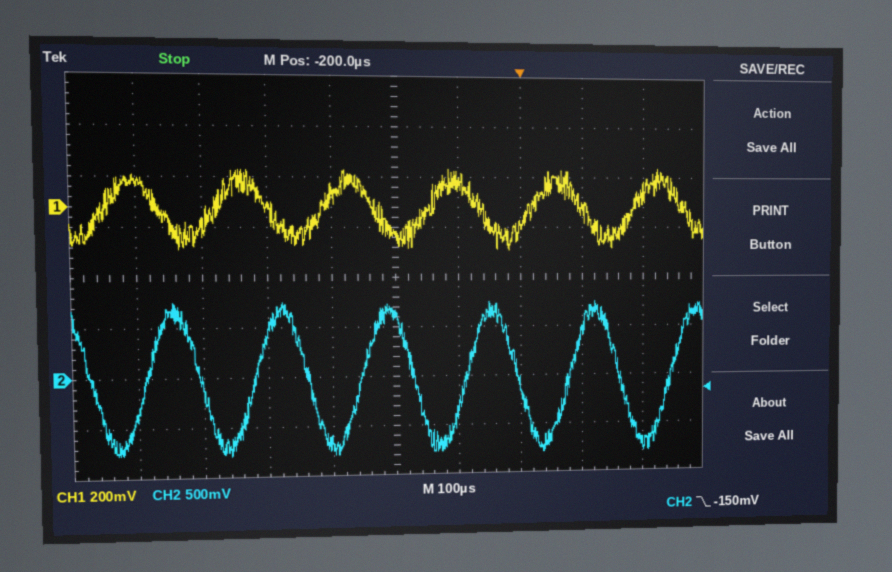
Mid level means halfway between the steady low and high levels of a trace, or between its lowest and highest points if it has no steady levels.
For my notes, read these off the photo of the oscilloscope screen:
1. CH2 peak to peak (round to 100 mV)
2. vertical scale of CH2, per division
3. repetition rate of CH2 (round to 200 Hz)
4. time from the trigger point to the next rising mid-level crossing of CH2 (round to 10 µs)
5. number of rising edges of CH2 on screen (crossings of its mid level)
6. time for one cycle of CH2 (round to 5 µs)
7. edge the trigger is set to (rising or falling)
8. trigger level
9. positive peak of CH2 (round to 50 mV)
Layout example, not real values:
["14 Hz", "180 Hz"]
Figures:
["1.50 V", "500 mV", "6.0 kHz", "80 µs", "6", "165 µs", "falling", "-150 mV", "750 mV"]
